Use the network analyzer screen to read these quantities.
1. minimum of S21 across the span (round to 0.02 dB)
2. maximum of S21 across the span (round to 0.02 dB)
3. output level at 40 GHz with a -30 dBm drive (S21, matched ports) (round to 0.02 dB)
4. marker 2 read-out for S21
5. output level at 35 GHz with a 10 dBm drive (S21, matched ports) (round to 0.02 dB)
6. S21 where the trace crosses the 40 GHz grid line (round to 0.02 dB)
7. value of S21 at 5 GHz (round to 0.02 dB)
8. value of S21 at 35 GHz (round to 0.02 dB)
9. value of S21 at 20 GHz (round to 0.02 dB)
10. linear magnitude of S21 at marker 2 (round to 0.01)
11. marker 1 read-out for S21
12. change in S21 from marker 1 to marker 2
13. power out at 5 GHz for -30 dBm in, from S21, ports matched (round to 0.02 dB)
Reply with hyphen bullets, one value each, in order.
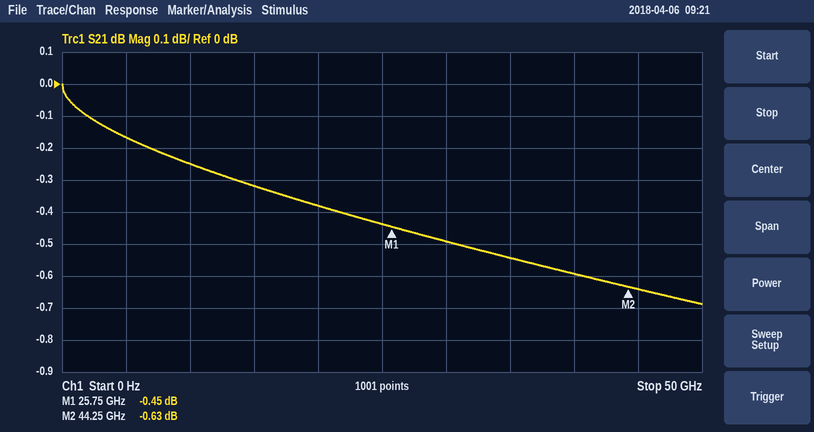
- -0.68 dB
- 0.00 dB
- -30.60 dBm
- -0.63 dB
- 9.46 dBm
- -0.60 dB
- -0.16 dB
- -0.54 dB
- -0.38 dB
- 0.93
- -0.45 dB
- -0.18 dB
- -30.16 dBm
